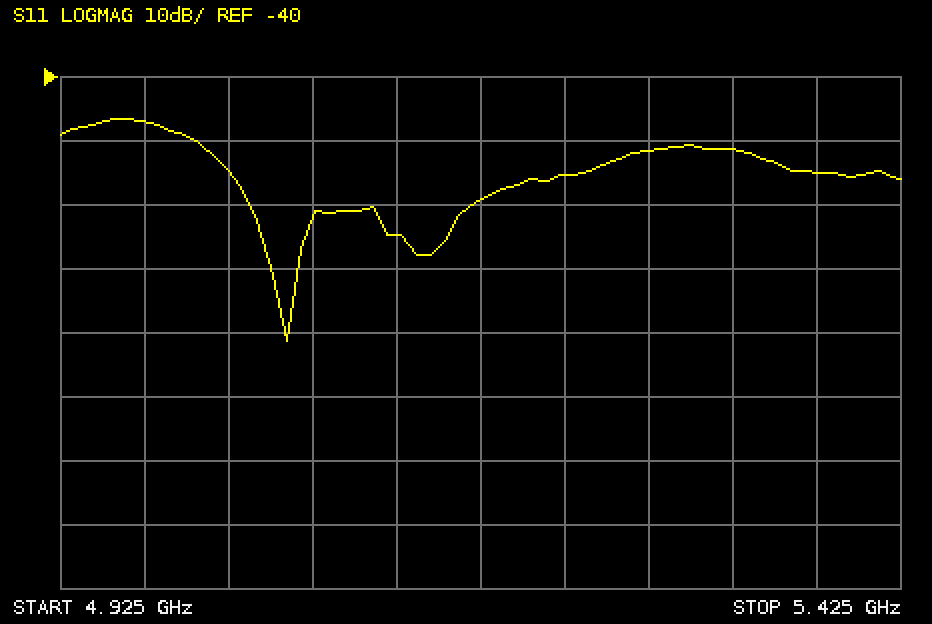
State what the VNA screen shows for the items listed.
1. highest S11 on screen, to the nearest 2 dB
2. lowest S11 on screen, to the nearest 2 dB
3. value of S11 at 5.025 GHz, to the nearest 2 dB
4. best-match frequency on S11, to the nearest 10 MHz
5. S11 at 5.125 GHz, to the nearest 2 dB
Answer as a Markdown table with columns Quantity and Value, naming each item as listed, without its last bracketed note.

| Quantity | Value |
|---|---|
| highest S11 on screen, to the nearest 2 dB | -46 dB |
| lowest S11 on screen, to the nearest 2 dB | -82 dB |
| value of S11 at 5.025 GHz, to the nearest 2 dB | -54 dB |
| best-match frequency on S11, to the nearest 10 MHz | 5.06 GHz |
| S11 at 5.125 GHz, to the nearest 2 dB | -64 dB |
